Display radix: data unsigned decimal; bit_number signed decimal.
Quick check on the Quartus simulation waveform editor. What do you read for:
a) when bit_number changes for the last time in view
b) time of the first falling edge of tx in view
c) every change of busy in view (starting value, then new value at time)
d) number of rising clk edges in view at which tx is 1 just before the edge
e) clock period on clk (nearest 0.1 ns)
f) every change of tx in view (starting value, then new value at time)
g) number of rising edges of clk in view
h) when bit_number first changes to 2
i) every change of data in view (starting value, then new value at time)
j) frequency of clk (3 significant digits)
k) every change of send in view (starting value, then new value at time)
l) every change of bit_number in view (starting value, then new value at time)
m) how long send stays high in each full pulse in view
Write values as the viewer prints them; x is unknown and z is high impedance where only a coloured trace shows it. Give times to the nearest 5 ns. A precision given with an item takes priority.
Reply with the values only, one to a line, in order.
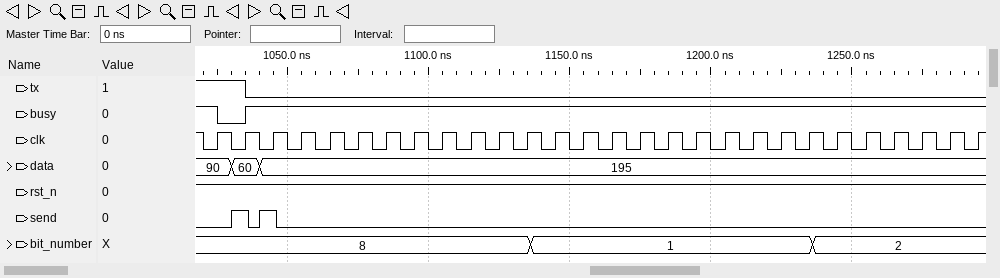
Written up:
1235 ns
1035 ns
1, 0 at 1025 ns, 1 at 1035 ns
2
10 ns
1, 0 at 1035 ns
28
1235 ns
90, 60 at 1030 ns, 195 at 1040 ns
100 MHz
0, 1 at 1030 ns, 0 at 1035 ns, 1 at 1040 ns, 0 at 1045 ns
8, 1 at 1135 ns, 2 at 1235 ns
5 ns, 5 ns
